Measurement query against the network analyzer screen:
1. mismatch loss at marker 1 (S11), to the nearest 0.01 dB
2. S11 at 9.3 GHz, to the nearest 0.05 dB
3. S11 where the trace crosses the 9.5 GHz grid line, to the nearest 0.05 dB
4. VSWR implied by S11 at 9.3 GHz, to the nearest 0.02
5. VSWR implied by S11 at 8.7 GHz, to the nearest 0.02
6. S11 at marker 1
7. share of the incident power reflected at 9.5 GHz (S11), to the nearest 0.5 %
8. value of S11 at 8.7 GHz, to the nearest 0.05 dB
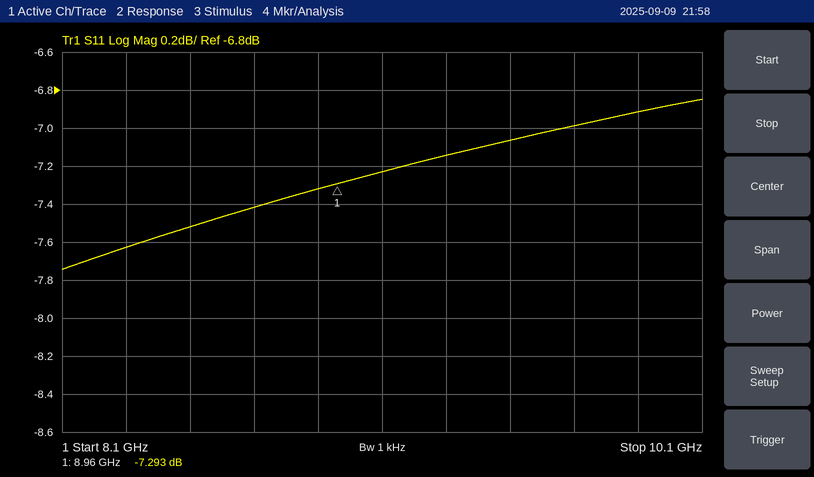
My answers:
0.90 dB
-7.15 dB
-7.05 dB
2.56
2.48
-7.293 dB
19.5 %
-7.40 dB
